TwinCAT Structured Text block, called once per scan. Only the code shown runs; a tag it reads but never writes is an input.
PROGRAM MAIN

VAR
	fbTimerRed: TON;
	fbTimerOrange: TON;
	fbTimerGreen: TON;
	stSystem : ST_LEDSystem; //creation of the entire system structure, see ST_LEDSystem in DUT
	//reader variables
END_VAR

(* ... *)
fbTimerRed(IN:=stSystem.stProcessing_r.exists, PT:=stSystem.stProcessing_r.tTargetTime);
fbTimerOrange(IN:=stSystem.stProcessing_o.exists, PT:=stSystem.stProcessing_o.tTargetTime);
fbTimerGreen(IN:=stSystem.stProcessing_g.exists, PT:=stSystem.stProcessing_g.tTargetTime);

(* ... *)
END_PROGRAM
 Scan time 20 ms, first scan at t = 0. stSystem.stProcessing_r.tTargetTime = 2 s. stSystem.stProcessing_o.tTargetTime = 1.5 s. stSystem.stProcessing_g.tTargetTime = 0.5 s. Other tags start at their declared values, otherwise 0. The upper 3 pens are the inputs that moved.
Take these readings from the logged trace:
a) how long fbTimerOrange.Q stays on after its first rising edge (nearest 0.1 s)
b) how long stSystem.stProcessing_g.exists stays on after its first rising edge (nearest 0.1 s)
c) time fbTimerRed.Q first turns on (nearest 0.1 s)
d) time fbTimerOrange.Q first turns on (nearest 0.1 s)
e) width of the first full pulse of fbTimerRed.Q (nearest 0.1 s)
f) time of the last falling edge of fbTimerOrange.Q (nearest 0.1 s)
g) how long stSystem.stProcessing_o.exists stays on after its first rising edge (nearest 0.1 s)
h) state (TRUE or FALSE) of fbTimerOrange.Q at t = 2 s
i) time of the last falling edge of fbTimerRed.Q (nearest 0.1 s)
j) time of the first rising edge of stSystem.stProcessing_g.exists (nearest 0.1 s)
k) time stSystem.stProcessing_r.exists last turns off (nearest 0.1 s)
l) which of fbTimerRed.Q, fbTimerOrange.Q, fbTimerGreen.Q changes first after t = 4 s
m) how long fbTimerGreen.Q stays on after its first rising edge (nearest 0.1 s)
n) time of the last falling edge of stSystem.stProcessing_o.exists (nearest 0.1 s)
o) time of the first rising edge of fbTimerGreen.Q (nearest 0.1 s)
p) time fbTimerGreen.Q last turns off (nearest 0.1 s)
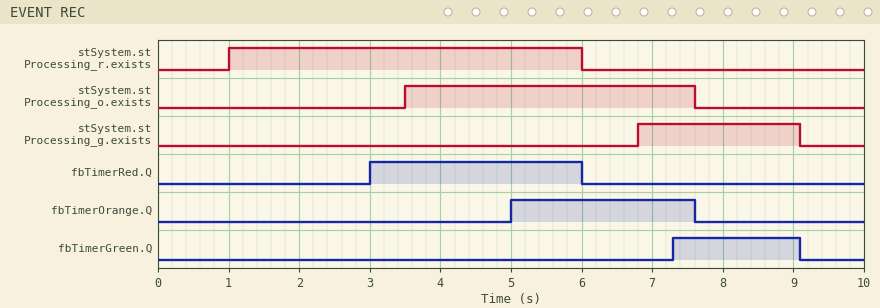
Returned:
2.6 s
2.3 s
3.0 s
5.0 s
3.0 s
7.6 s
4.1 s
FALSE
6.0 s
6.8 s
6.0 s
fbTimerOrange.Q
1.8 s
7.6 s
7.3 s
9.1 s
